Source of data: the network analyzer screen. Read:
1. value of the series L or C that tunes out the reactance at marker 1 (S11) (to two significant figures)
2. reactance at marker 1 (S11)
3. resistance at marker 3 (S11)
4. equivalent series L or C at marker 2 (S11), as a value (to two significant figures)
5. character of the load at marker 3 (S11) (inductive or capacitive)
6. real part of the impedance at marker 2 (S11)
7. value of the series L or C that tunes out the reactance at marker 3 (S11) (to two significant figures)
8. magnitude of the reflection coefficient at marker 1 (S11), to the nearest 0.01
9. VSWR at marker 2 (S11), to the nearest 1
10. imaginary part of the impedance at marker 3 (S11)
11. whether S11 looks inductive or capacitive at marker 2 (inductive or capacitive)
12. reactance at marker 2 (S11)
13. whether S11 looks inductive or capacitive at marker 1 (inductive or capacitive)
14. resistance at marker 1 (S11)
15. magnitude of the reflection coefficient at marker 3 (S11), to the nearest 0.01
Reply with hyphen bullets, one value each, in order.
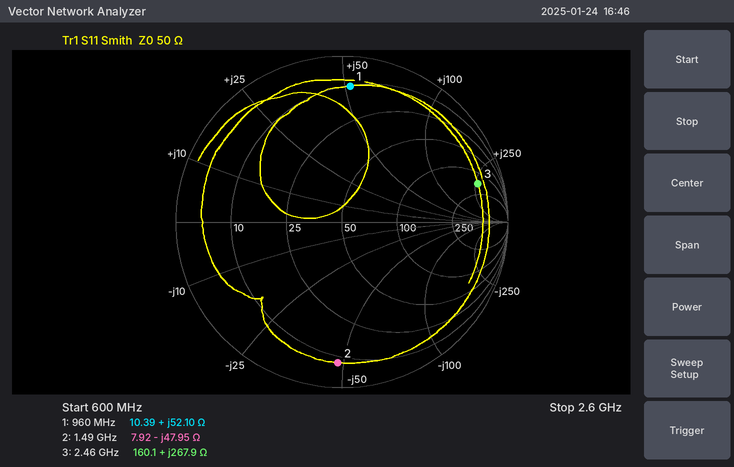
- 3.2 pF
- +52.10 Ω
- 160.1 Ω
- 2.2 pF
- inductive
- 7.92 Ω
- 240 fF
- 0.82
- 12
- +267.9 Ω
- capacitive
- -47.95 Ω
- inductive
- 10.39 Ω
- 0.85
